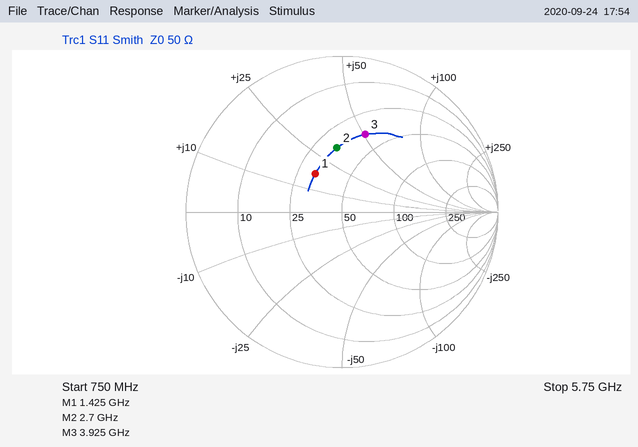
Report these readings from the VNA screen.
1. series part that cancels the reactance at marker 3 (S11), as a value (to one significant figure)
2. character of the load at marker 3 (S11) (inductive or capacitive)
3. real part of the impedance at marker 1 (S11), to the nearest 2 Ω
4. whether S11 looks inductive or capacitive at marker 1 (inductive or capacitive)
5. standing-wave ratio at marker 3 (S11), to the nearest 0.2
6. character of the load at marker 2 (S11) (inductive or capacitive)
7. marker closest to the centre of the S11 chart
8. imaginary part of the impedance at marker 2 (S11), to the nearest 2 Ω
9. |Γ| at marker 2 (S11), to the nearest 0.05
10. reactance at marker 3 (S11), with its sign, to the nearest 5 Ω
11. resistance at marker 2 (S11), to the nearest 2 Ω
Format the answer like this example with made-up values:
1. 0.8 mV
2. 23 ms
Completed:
1. 800 fF
2. inductive
3. 32 Ω
4. inductive
5. 3.2
6. inductive
7. marker 1
8. +34 Ω
9. 0.40
10. +50 Ω
11. 34 Ω
